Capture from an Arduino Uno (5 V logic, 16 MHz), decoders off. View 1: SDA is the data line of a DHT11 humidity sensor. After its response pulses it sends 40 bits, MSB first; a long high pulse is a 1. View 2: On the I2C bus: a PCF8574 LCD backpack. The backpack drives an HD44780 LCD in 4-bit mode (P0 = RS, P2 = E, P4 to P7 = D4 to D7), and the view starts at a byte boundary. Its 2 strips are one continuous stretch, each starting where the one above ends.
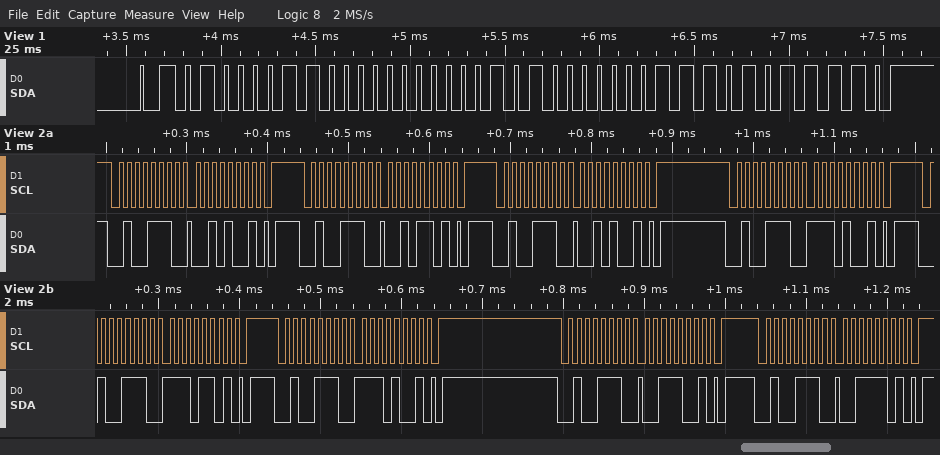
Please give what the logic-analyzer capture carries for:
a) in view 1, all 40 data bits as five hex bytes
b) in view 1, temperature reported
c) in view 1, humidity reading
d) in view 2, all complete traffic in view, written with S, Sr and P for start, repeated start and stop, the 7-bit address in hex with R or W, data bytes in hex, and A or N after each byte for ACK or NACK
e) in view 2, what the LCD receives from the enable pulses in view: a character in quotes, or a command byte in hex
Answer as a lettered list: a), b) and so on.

a) 43 00 14 07 5E
b) 20.7 °C
c) 67 %
d) S 27W A 29 A P S 27W A 2D A P S 27W A 29 A P S 27W A E9 A P S 27W A ED A P S 27W A E9 A P S 27W A 39 A P S 27W A 3D A P
e) '.'
